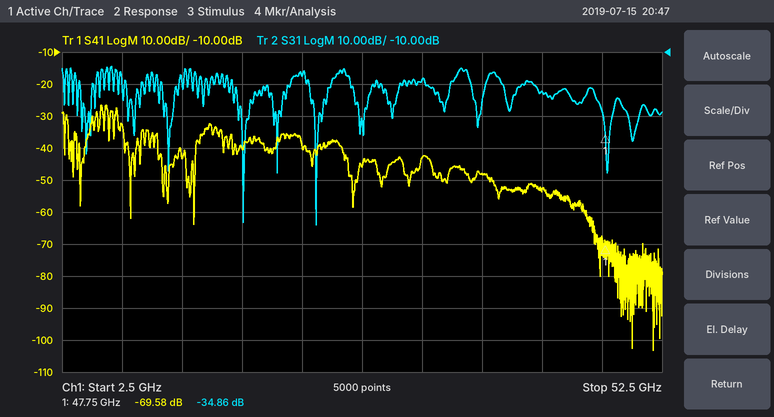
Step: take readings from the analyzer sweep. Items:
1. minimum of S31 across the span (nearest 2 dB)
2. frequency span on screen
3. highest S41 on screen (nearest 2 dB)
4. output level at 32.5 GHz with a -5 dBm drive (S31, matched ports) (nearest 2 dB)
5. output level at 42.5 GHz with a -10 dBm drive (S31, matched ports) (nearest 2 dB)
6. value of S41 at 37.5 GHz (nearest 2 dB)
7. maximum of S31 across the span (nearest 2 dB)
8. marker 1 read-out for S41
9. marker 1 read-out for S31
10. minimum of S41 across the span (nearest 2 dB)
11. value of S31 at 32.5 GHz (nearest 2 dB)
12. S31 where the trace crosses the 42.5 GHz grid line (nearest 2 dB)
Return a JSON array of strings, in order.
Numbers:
["-64 dB", "50 GHz", "-26 dB", "-24 dBm", "-32 dBm", "-48 dB", "-14 dB", "-69.58 dB", "-34.86 dB", "-104 dB", "-18 dB", "-22 dB"]
